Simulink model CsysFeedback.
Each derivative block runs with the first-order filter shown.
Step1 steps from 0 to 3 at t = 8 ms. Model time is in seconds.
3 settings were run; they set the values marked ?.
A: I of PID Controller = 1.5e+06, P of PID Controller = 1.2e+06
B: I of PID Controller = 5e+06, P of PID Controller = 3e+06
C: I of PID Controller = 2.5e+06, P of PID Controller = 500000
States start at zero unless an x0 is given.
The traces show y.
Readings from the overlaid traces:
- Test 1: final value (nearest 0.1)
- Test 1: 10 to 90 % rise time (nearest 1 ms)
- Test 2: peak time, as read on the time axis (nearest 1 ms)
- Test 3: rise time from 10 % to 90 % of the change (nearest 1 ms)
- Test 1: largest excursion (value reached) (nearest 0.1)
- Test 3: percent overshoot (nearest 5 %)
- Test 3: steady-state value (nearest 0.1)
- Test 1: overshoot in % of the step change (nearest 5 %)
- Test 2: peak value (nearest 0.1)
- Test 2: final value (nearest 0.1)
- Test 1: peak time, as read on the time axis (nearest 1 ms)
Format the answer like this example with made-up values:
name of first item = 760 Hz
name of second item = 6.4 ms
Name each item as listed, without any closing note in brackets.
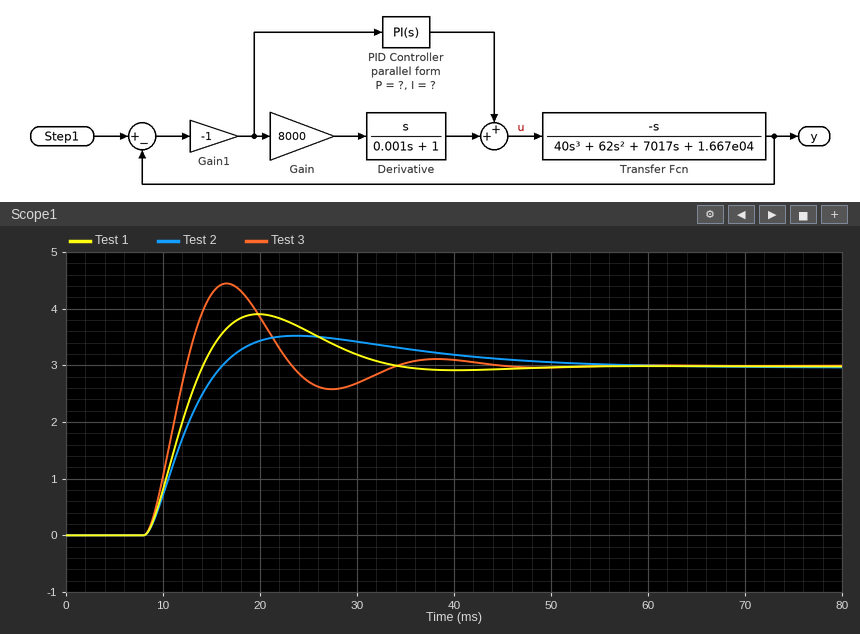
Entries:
Test 1: final value = 3.0
Test 1: 10 to 90 % rise time = 4 ms
Test 2: peak time, as read on the time axis = 24 ms
Test 3: rise time from 10 % to 90 % of the change = 3 ms
Test 1: largest excursion (value reached) = 3.9
Test 3: percent overshoot = 50 %
Test 3: steady-state value = 3.0
Test 1: overshoot in % of the step change = 30 %
Test 2: peak value = 3.5
Test 2: final value = 3.0
Test 1: peak time, as read on the time axis = 20 ms
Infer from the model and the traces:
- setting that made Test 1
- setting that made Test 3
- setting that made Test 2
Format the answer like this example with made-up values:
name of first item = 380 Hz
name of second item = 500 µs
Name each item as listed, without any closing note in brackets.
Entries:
setting that made Test 1 = A
setting that made Test 3 = B
setting that made Test 2 = C
